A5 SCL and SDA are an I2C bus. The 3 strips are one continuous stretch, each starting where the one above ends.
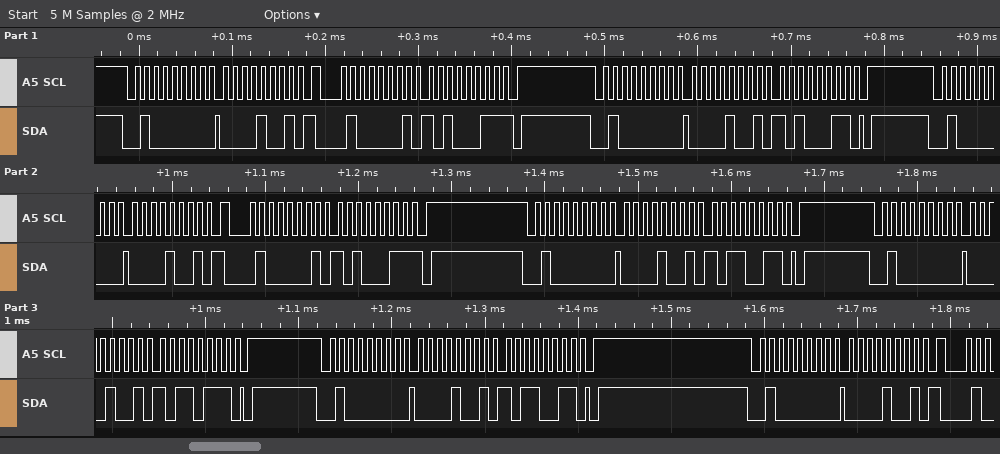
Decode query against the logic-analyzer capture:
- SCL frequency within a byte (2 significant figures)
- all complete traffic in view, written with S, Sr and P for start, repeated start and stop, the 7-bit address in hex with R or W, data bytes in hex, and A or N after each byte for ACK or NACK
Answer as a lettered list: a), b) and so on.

a) 100 kHz
b) S 20W A 09 A Sr 20R A A3 N P S 20W A 09 A A3 A P S 20W A 09 A Sr 20R A A3 N P S 20W A 09 A B3 A P S 20W A 09 A B7 A P S 20W A 09 A B3 A P S 20W A 09 A
